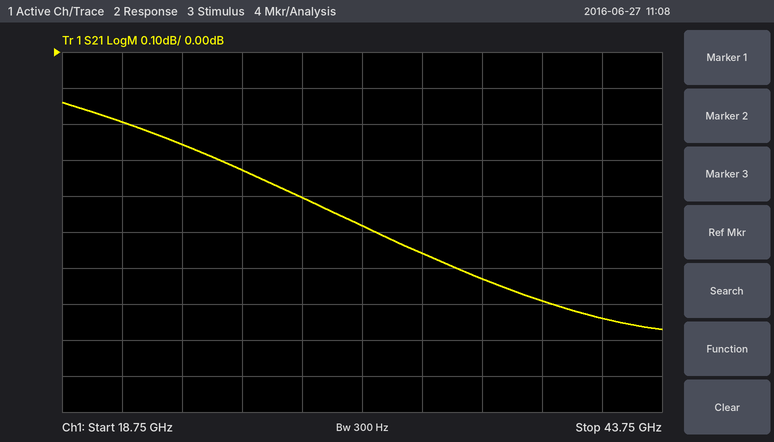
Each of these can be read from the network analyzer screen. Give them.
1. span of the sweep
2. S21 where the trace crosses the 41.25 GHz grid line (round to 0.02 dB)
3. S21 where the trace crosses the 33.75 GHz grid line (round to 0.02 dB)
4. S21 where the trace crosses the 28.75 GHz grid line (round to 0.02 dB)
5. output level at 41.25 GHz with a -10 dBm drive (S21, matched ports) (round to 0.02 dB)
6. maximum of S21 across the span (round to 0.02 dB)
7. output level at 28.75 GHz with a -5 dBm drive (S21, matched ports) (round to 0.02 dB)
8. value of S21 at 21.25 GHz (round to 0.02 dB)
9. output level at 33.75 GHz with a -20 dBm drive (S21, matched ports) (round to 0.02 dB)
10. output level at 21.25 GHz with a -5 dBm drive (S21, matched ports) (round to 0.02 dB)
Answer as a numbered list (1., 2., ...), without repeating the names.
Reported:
1. 25 GHz
2. -0.74 dB
3. -0.56 dB
4. -0.40 dB
5. -10.74 dBm
6. -0.14 dB
7. -5.40 dBm
8. -0.20 dB
9. -20.56 dBm
10. -5.20 dBm
